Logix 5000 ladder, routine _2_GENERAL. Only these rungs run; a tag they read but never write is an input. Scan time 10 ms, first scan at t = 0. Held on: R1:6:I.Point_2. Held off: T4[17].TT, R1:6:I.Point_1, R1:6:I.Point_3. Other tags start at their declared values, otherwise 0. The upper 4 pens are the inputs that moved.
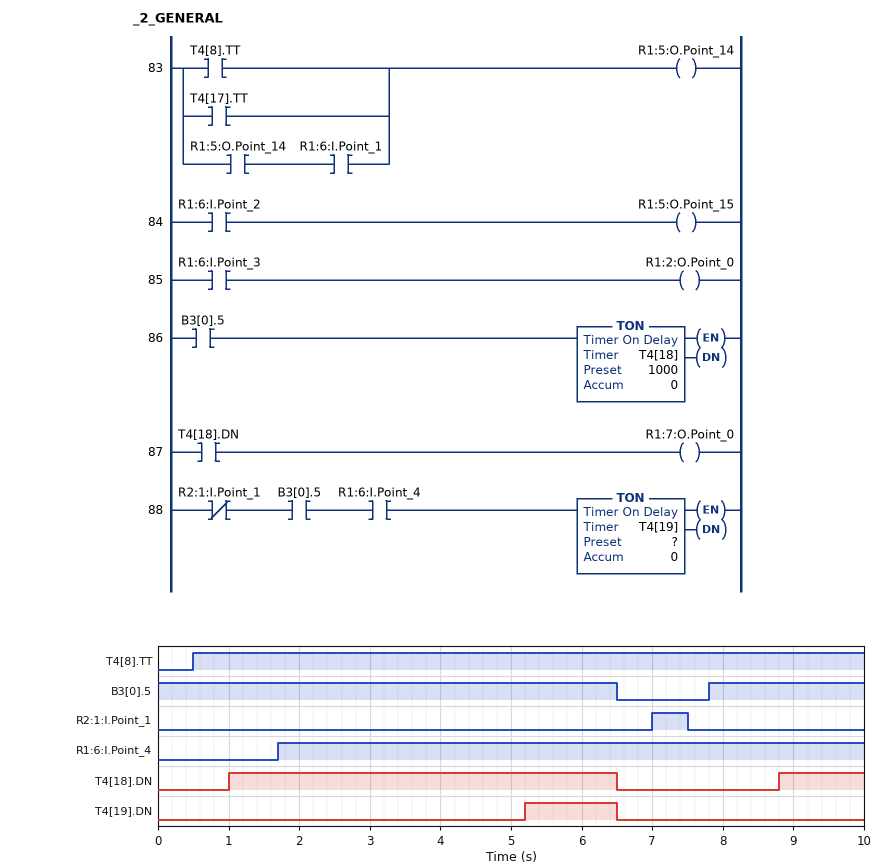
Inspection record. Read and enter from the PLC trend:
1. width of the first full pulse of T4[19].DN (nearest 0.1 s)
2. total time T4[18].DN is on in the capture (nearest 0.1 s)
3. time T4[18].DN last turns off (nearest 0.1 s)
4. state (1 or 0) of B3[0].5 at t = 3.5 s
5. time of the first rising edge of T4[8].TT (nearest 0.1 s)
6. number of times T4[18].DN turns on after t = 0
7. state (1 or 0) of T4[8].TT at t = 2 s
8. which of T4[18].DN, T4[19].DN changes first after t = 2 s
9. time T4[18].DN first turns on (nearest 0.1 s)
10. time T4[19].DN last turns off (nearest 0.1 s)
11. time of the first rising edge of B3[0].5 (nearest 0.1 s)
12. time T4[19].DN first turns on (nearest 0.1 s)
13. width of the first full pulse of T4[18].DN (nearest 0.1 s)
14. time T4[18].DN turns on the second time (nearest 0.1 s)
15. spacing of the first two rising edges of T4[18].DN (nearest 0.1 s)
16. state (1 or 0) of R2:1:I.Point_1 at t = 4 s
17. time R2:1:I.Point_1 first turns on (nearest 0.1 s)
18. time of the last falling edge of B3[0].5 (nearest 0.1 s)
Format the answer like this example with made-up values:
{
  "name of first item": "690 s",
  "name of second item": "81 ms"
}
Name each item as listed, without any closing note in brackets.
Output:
{
  "width of the first full pulse of T4[19].DN": "1.3 s",
  "total time T4[18].DN is on in the capture": "6.7 s",
  "time T4[18].DN last turns off": "6.5 s",
  "state (1 or 0) of B3[0].5 at t = 3.5 s": "1",
  "time of the first rising edge of T4[8].TT": "0.5 s",
  "number of times T4[18].DN turns on after t = 0": "2",
  "state (1 or 0) of T4[8].TT at t = 2 s": "1",
  "which of T4[18].DN, T4[19].DN changes first after t = 2 s": "T4[19].DN",
  "time T4[18].DN first turns on": "1.0 s",
  "time T4[19].DN last turns off": "6.5 s",
  "time of the first rising edge of B3[0].5": "7.8 s",
  "time T4[19].DN first turns on": "5.2 s",
  "width of the first full pulse of T4[18].DN": "5.5 s",
  "time T4[18].DN turns on the second time": "8.8 s",
  "spacing of the first two rising edges of T4[18].DN": "7.8 s",
  "state (1 or 0) of R2:1:I.Point_1 at t = 4 s": "0",
  "time R2:1:I.Point_1 first turns on": "7.0 s",
  "time of the last falling edge of B3[0].5": "6.5 s"
}
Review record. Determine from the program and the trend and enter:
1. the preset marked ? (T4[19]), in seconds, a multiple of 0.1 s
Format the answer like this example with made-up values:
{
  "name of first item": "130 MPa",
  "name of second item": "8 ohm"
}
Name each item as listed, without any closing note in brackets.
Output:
{
  "the preset marked ? (T4[19]), in seconds, a multiple of 0.1 s": "3.5 s"
}
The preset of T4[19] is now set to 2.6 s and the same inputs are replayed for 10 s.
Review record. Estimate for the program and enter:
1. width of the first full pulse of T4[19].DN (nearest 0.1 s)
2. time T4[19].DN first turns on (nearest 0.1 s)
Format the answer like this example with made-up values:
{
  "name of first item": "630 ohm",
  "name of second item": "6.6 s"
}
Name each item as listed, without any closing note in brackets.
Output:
{
  "width of the first full pulse of T4[19].DN": "2.2 s",
  "time T4[19].DN first turns on": "4.3 s"
}
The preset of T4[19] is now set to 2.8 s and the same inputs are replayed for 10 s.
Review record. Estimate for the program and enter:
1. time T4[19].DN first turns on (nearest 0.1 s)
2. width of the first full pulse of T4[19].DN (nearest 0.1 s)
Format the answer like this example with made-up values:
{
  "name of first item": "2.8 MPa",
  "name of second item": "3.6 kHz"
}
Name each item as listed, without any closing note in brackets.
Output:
{
  "time T4[19].DN first turns on": "4.5 s",
  "width of the first full pulse of T4[19].DN": "2.0 s"
}
